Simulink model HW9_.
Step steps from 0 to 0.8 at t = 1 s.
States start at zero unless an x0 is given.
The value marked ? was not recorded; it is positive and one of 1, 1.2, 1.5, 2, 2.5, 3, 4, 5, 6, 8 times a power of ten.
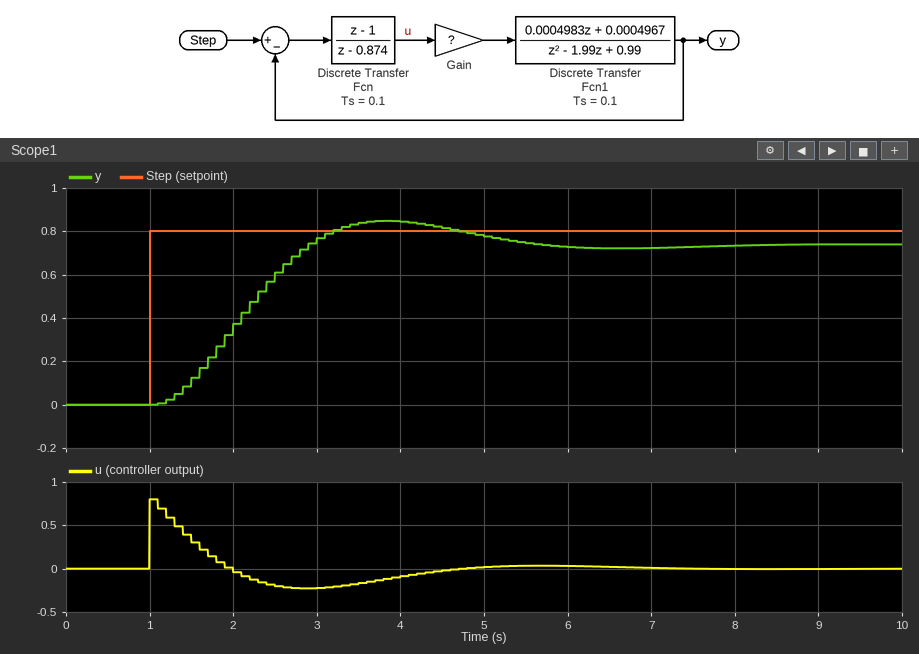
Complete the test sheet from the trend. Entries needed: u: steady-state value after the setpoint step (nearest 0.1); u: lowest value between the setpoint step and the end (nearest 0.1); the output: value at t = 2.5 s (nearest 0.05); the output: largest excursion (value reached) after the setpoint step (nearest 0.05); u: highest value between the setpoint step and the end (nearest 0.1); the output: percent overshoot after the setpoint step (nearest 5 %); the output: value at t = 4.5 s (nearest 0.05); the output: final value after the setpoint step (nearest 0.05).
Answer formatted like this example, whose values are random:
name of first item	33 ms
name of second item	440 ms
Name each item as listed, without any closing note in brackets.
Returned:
u: steady-state value after the setpoint step	0.0
u: lowest value between the setpoint step and the end	-0.2
the output: value at t = 2.5 s	0.60
the output: largest excursion (value reached) after the setpoint step	0.85
u: highest value between the setpoint step and the end	0.8
the output: percent overshoot after the setpoint step	15 %
the output: value at t = 4.5 s	0.80
the output: final value after the setpoint step	0.75
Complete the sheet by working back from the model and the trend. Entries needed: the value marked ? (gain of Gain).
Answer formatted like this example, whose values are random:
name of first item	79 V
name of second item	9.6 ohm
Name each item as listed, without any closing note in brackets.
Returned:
the value marked ?	15
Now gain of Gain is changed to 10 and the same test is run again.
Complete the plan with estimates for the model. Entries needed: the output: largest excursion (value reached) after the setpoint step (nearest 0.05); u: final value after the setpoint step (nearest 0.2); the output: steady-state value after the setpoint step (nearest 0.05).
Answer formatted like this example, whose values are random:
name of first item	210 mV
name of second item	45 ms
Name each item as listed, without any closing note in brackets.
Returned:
the output: largest excursion (value reached) after the setpoint step	0.75
u: final value after the setpoint step	0.0
the output: steady-state value after the setpoint step	0.70
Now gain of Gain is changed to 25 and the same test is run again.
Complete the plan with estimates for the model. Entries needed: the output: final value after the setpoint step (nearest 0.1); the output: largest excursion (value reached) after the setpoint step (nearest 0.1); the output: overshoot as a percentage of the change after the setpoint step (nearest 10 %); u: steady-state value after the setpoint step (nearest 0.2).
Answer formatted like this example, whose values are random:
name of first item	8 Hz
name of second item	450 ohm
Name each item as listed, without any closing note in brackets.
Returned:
the output: final value after the setpoint step	0.8
the output: largest excursion (value reached) after the setpoint step	1.0
the output: overshoot as a percentage of the change after the setpoint step	30 %
u: steady-state value after the setpoint step	0.0
